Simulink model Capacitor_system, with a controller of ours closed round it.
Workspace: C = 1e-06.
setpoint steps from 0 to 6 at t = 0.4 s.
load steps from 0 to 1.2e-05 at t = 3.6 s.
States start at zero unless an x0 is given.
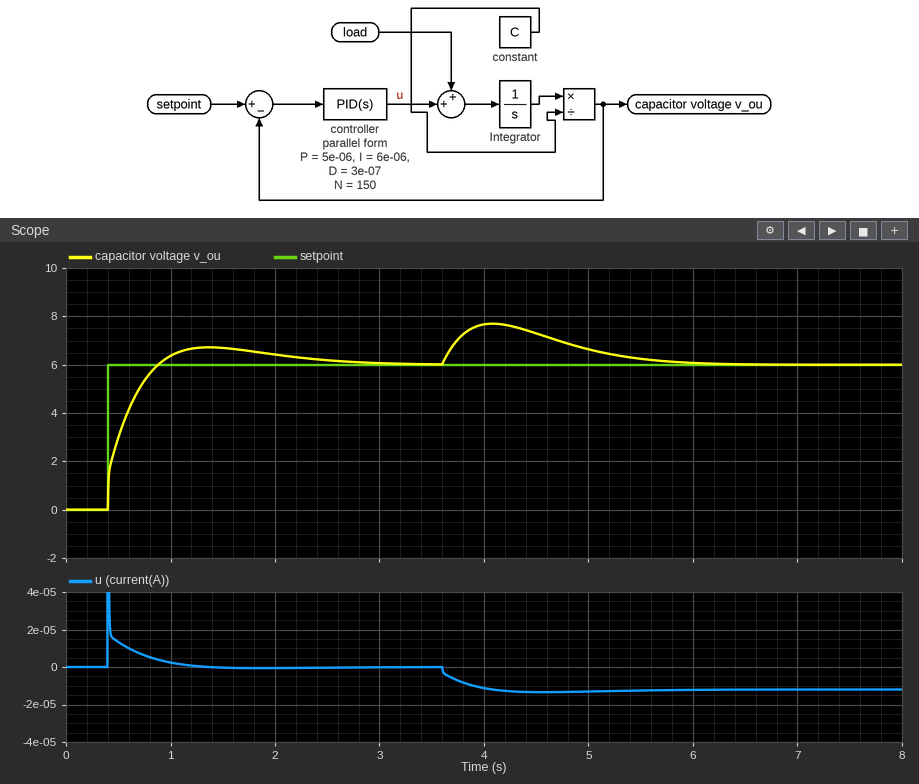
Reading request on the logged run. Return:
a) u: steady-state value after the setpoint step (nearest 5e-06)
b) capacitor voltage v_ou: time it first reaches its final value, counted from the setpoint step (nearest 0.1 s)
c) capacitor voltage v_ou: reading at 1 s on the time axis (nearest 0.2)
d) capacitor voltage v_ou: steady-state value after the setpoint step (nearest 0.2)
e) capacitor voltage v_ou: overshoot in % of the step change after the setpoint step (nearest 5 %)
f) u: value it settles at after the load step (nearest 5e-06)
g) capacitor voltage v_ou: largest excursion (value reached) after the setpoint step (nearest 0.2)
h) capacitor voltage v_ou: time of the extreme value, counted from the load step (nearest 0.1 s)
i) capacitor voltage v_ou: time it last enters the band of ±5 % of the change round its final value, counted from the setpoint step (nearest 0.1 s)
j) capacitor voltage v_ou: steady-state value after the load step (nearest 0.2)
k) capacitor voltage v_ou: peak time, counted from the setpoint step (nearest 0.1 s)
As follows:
0.000000
0.5 s
6.4
6.0
10 %
-0.000010
6.8
0.5 s
1.8 s
6.0
1.0 s
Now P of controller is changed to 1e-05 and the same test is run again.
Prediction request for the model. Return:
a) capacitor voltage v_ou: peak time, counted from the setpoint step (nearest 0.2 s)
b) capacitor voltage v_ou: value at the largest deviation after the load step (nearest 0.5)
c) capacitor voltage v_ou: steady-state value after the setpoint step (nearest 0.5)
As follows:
0.8 s
7.0
6.0
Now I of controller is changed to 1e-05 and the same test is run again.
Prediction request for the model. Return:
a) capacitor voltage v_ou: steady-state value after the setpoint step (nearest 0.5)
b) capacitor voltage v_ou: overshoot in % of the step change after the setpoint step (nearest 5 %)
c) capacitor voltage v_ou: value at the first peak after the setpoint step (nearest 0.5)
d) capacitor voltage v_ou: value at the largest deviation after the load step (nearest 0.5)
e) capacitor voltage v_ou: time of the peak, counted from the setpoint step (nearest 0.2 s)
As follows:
6.0
15 %
7.0
7.5
0.8 s
